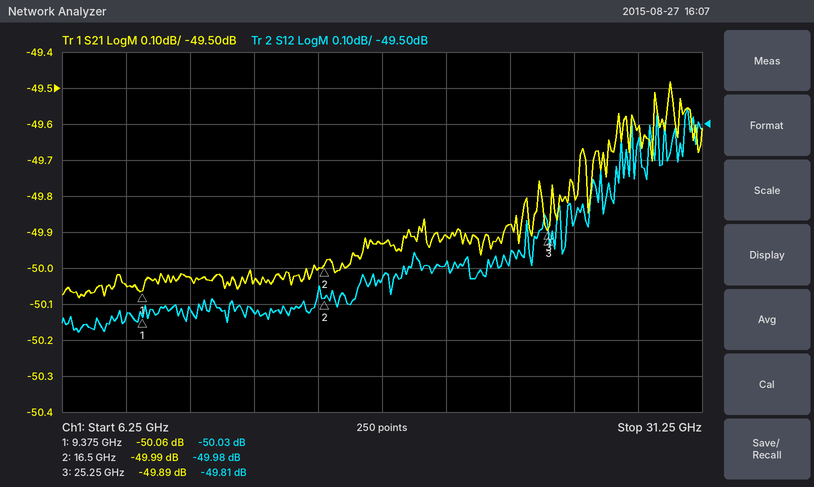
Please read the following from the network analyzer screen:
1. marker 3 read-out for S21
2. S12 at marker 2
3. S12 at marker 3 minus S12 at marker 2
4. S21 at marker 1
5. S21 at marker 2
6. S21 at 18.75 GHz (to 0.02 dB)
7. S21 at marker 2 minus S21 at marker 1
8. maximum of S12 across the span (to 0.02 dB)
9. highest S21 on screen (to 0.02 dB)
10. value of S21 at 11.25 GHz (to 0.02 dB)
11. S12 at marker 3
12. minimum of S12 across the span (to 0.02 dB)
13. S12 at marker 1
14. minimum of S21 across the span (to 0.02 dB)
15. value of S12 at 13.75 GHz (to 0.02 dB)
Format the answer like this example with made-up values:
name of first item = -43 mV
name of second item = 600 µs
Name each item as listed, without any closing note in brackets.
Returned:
marker 3 read-out for S21 = -49.89 dB
S12 at marker 2 = -49.98 dB
S12 at marker 3 minus S12 at marker 2 = 0.17 dB
S21 at marker 1 = -50.06 dB
S21 at marker 2 = -49.99 dB
S21 at 18.75 GHz = -49.94 dB
S21 at marker 2 minus S21 at marker 1 = 0.07 dB
maximum of S12 across the span = -49.46 dB
highest S21 on screen = -49.48 dB
value of S21 at 11.25 GHz = -50.02 dB
S12 at marker 3 = -49.81 dB
minimum of S12 across the span = -50.08 dB
S12 at marker 1 = -50.03 dB
minimum of S21 across the span = -50.08 dB
value of S12 at 13.75 GHz = -50.02 dB
